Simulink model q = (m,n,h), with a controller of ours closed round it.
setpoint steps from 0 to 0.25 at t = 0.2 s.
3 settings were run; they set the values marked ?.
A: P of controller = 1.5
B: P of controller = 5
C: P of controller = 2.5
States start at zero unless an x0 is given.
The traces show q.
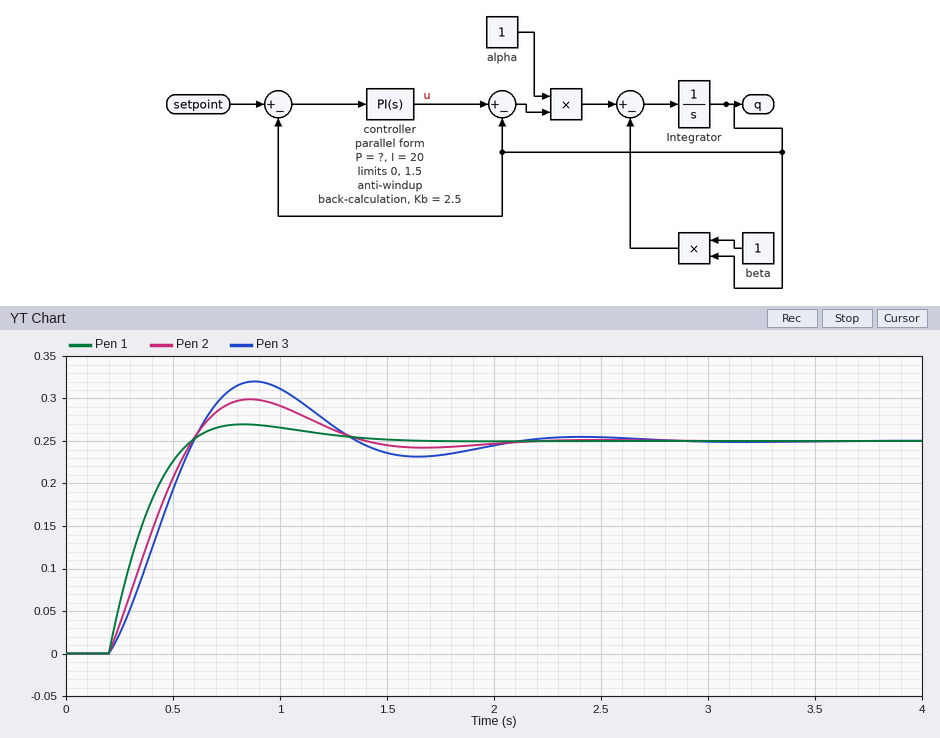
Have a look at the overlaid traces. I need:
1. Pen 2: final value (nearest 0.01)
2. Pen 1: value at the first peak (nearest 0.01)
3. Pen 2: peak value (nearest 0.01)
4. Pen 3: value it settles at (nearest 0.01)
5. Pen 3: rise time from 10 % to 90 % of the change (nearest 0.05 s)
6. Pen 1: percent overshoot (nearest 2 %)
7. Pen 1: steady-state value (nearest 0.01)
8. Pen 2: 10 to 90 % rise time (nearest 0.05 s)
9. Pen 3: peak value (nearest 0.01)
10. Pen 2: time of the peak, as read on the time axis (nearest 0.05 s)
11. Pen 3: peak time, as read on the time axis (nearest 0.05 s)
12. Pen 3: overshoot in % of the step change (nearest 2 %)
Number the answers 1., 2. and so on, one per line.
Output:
1. 0.25
2. 0.27
3. 0.30
4. 0.25
5. 0.30 s
6. 8 %
7. 0.25
8. 0.30 s
9. 0.32
10. 0.85 s
11. 0.90 s
12. 28 %
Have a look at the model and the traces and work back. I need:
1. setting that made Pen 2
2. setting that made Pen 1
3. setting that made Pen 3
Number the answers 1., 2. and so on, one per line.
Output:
1. C
2. B
3. A
